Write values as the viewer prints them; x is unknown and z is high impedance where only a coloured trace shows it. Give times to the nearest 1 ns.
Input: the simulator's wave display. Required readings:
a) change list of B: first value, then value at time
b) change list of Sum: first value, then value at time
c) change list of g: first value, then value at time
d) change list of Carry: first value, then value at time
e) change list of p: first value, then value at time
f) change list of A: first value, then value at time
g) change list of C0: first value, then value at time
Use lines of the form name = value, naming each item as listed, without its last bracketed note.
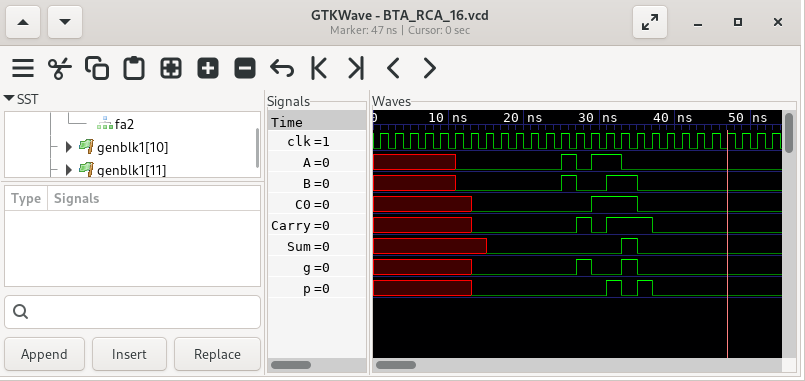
change list of B: first value, then value at time = x, 0 at 11 ns, 1 at 25 ns, 0 at 27 ns, 1 at 31 ns, 0 at 35 ns
change list of Sum: first value, then value at time = x, 0 at 15 ns, 1 at 33 ns, 0 at 35 ns
change list of g: first value, then value at time = x, 0 at 13 ns, 1 at 27 ns, 0 at 29 ns, 1 at 33 ns, 0 at 35 ns
change list of Carry: first value, then value at time = x, 0 at 13 ns, 1 at 27 ns, 0 at 29 ns, 1 at 31 ns, 0 at 37 ns
change list of p: first value, then value at time = x, 0 at 13 ns, 1 at 31 ns, 0 at 33 ns, 1 at 35 ns, 0 at 37 ns
change list of A: first value, then value at time = x, 0 at 11 ns, 1 at 25 ns, 0 at 27 ns, 1 at 29 ns, 0 at 33 ns
change list of C0: first value, then value at time = x, 0 at 13 ns, 1 at 29 ns, 0 at 35 ns
